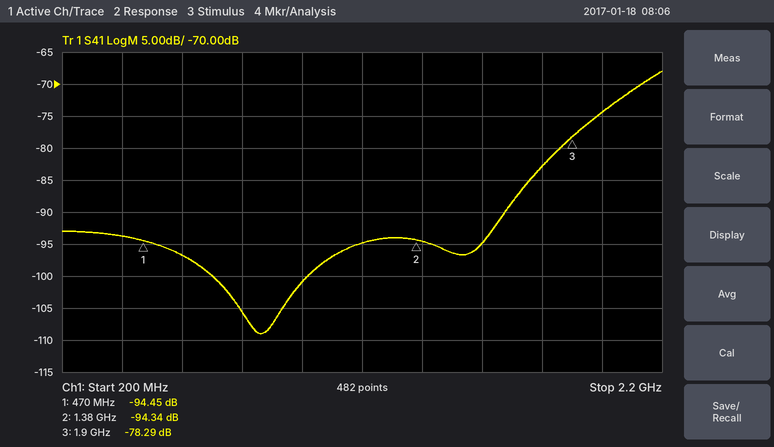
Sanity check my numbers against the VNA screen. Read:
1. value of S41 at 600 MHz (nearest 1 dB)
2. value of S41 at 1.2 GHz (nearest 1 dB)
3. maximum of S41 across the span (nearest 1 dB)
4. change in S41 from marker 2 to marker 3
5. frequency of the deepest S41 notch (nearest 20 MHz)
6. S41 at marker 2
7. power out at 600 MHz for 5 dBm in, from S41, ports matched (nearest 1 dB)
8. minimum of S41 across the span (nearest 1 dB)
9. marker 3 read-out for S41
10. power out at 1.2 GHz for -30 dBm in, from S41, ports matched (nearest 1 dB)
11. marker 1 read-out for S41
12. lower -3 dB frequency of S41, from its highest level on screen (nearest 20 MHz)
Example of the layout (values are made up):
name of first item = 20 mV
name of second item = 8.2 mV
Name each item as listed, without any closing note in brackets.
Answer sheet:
value of S41 at 600 MHz = -97 dB
value of S41 at 1.2 GHz = -95 dB
maximum of S41 across the span = -68 dB
change in S41 from marker 2 to marker 3 = 16.05 dB
frequency of the deepest S41 notch = 860 MHz
S41 at marker 2 = -94.34 dB
power out at 600 MHz for 5 dBm in, from S41, ports matched = -92 dBm
minimum of S41 across the span = -109 dB
marker 3 read-out for S41 = -78.29 dB
power out at 1.2 GHz for -30 dBm in, from S41, ports matched = -125 dBm
marker 1 read-out for S41 = -94.45 dB
lower -3 dB frequency of S41, from its highest level on screen = 2.10 GHz
